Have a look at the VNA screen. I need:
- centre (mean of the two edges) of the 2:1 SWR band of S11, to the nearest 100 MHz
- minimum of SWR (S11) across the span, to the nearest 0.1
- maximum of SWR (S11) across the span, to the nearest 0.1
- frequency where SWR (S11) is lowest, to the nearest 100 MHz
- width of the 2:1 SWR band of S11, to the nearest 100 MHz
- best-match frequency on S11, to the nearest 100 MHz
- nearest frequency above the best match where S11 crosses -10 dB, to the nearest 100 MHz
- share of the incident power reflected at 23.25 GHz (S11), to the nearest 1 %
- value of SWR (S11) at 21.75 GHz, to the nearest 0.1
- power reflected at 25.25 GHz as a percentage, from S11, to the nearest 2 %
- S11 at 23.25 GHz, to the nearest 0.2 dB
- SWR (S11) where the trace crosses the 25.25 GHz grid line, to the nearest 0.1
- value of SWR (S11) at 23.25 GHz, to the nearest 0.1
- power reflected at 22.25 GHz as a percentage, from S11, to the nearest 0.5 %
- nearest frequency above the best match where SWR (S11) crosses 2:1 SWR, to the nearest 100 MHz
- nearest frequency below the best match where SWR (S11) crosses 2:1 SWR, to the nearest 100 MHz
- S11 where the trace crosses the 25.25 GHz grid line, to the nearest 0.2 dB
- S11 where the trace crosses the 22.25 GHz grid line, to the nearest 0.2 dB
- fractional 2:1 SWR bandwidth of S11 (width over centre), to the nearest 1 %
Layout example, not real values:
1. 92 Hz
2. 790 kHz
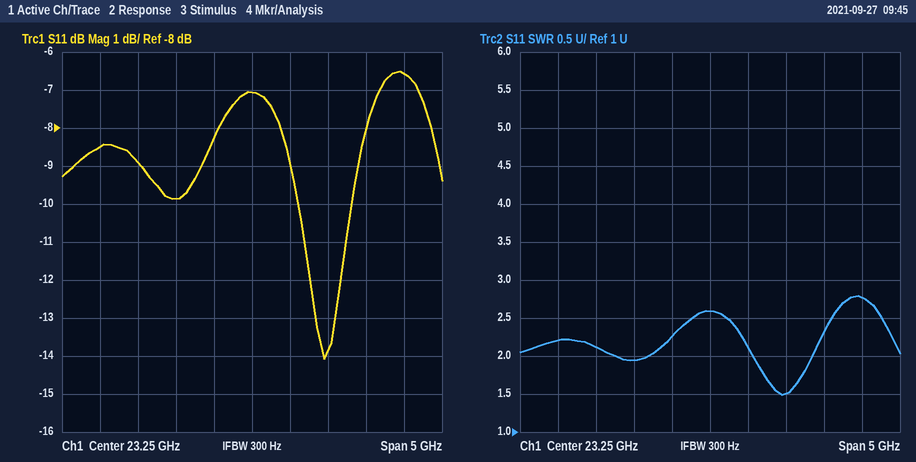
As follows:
1. 24.2 GHz
2. 1.5
3. 2.8
4. 24.2 GHz
5. 800 MHz
6. 24.2 GHz
7. 24.6 GHz
8. 20 %
9. 2.1
10. 22 %
11. -7.0 dB
12. 2.8
13. 2.6
14. 10.5 %
15. 24.6 GHz
16. 23.8 GHz
17. -6.6 dB
18. -9.8 dB
19. 3 %
